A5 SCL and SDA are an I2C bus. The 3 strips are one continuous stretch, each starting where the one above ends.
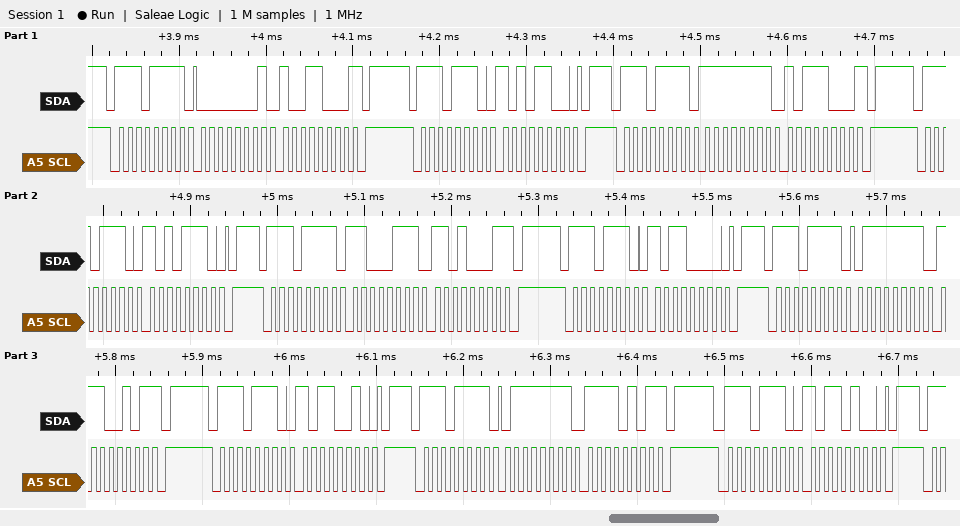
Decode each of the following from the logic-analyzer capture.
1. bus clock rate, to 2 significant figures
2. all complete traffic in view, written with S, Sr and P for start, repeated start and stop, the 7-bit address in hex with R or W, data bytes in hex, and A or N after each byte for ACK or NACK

100 kHz
S 77R A 01 A 98 N P S 77W A AC A P S 77R A FF A B8 N P S 77W A AE A P S 77R A C7 A D1 N P S 77W A B0 A P S 77R A 7F A E5 N P S 77W A B2 A P S 77R A 7F A F5 N P S 77W A B4 A P
